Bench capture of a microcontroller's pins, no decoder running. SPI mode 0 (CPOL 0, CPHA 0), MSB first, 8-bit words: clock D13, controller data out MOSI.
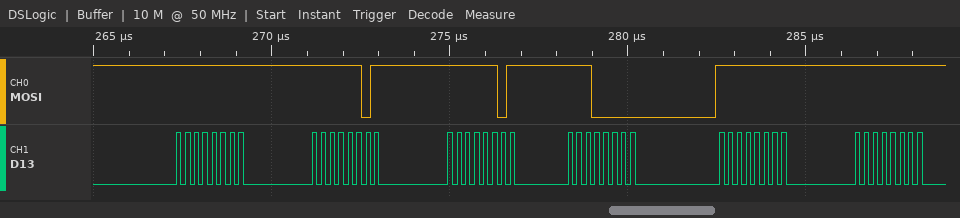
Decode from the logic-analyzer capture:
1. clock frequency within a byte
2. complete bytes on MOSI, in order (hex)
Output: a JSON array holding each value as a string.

["4 MHz", "FF FD FD E0 FF FF"]
